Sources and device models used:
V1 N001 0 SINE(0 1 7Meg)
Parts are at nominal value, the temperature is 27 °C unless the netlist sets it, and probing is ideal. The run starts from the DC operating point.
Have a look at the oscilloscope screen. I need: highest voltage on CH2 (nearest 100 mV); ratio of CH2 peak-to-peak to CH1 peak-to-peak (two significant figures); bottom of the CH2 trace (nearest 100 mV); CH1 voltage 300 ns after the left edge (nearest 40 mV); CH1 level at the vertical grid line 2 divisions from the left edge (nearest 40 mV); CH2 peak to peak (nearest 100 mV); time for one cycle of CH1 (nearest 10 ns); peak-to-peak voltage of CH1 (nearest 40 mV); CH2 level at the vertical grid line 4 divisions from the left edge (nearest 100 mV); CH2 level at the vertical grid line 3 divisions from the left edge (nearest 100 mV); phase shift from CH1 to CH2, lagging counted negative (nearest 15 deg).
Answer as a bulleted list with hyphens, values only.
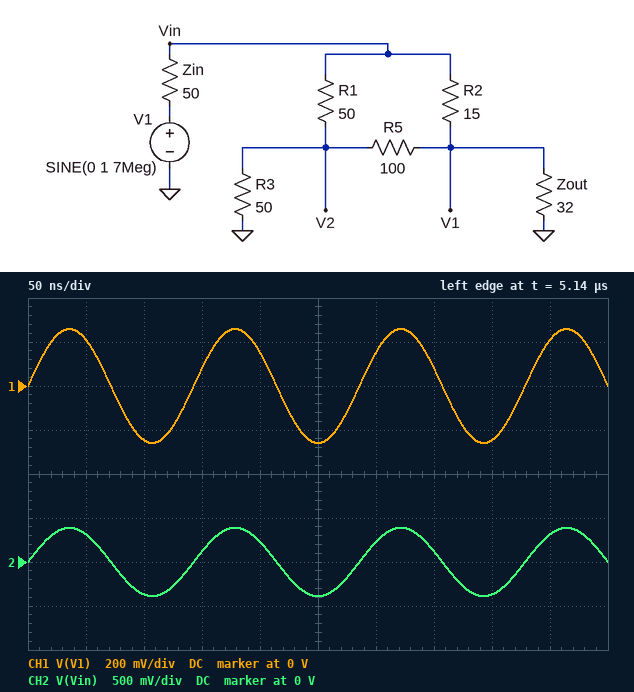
- 400 mV
- 1.5
- -400 mV
- 160 mV
- -240 mV
- 800 mV
- 140 ns
- 520 mV
- 200 mV
- 100 mV
- 0 deg
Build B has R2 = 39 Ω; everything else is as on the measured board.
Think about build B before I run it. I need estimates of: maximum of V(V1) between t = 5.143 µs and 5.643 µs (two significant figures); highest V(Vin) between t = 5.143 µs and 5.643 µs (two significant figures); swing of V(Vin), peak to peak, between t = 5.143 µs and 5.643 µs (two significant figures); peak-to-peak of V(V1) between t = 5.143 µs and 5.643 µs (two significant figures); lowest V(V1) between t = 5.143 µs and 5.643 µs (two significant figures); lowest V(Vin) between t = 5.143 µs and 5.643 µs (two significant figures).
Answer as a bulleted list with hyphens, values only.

- 210 mV
- 450 mV
- 910 mV
- 410 mV
- -210 mV
- -450 mV
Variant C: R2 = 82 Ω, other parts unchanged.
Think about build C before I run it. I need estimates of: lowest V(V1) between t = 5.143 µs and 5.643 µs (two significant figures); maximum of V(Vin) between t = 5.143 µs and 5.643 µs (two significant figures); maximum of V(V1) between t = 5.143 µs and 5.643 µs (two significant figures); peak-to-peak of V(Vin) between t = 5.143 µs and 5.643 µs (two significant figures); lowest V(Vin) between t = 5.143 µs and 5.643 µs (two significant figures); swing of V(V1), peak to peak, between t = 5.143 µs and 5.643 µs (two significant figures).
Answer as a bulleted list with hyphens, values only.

- -160 mV
- 510 mV
- 160 mV
- 1.0 V
- -510 mV
- 320 mV
